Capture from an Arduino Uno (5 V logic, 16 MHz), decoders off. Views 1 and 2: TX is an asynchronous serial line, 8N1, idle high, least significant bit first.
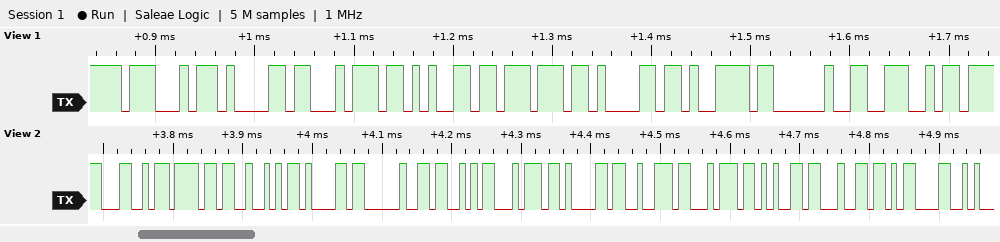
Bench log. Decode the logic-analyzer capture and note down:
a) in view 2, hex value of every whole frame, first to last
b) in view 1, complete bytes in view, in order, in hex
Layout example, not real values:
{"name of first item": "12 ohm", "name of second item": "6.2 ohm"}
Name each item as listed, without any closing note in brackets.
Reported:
{"in view 2, hex value of every whole frame, first to last": "4C 6F 52 61 20 53 74 61 72 74 65 64 0D", "in view 1, complete bytes in view, in order, in hex": "0x47 0x61 0x74 0x65 0x77 0x61 0x79 0x20 0x4E"}
